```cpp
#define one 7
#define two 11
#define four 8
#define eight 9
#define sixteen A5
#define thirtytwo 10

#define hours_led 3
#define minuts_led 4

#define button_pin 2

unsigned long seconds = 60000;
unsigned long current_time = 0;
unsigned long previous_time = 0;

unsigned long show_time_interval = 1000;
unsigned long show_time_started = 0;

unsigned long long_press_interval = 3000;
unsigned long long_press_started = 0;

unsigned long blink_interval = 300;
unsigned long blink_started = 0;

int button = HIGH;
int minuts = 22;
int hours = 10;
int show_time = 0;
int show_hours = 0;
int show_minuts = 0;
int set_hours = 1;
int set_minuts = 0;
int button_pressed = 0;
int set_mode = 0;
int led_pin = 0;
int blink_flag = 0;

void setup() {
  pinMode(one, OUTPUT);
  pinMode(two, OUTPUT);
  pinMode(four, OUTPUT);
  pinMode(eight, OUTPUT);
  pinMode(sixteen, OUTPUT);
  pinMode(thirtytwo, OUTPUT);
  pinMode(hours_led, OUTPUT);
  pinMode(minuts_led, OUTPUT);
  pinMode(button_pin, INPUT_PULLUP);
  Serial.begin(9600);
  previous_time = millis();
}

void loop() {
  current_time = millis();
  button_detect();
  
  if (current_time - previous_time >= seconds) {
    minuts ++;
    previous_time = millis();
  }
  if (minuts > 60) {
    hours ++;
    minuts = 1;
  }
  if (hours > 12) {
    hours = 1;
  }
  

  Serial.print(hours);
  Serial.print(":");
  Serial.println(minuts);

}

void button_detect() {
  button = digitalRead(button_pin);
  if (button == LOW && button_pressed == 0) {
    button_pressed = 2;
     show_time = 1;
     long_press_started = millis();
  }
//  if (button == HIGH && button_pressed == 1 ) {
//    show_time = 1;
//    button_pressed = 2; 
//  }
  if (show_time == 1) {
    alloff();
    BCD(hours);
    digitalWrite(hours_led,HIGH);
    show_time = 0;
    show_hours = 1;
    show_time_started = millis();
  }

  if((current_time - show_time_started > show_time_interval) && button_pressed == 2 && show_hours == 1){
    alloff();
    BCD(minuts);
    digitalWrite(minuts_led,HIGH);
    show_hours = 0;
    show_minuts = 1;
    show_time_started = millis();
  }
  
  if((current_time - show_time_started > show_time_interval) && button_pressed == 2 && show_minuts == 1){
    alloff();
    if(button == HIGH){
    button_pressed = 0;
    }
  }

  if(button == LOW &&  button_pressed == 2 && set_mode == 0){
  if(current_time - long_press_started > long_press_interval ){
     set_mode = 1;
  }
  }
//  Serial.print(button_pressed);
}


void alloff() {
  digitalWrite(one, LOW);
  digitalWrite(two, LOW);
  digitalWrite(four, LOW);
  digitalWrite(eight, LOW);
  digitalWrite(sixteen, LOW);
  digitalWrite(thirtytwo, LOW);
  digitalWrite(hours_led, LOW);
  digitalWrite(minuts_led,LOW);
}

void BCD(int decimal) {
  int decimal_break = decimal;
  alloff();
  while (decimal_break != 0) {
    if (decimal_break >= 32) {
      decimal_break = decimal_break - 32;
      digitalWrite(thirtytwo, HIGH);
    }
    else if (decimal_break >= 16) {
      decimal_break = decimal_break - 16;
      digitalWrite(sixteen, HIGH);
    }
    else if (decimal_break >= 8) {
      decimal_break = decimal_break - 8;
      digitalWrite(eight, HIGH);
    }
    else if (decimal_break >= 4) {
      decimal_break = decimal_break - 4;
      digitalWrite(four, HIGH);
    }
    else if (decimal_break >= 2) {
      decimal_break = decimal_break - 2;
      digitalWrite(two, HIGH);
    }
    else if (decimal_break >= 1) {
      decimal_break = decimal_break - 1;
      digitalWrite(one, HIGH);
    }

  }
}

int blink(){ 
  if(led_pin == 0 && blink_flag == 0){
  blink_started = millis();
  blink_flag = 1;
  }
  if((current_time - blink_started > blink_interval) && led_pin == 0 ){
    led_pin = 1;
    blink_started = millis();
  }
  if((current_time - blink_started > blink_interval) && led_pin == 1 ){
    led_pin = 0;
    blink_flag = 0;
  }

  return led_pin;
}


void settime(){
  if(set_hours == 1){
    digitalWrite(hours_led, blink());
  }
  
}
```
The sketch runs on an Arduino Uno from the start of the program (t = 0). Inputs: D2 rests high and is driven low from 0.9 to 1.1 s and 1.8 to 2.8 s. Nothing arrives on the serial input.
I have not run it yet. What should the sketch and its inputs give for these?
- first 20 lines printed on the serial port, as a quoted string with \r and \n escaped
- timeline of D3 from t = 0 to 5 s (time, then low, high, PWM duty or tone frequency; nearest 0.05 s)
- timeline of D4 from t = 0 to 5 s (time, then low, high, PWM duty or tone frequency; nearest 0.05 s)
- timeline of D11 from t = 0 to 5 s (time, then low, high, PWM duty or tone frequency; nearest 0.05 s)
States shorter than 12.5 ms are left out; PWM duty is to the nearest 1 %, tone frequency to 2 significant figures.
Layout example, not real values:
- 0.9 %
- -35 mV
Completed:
- "10:22\r\n10:22\r\n10:22\r\n10:22\r\n10:22\r\n10:22\r\n10:22\r\n10:22\r\n10:22\r\n10:22\r\n10:22\r\n10:22\r\n10:22\r\n10:22\r\n10:22\r\n10:22\r\n10:22\r\n10:22\r\n10:22\r\n10:22\r\n"
- 0 s low; 0.9 s high; 1.9 s low
- 0 s low; 1.9 s high; 2.9 s low
- 0 s low; 0.9 s high; 2.9 s low
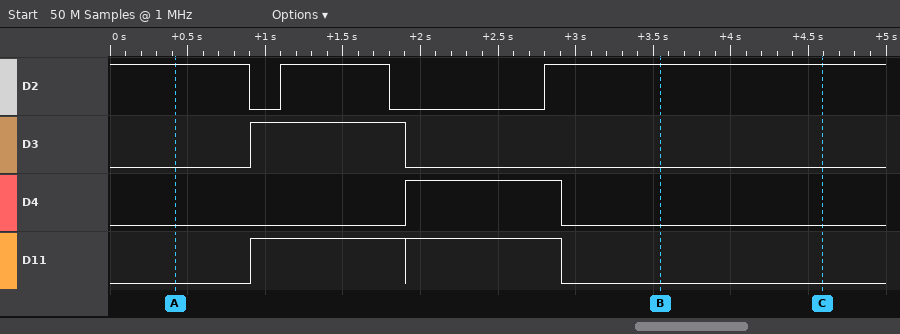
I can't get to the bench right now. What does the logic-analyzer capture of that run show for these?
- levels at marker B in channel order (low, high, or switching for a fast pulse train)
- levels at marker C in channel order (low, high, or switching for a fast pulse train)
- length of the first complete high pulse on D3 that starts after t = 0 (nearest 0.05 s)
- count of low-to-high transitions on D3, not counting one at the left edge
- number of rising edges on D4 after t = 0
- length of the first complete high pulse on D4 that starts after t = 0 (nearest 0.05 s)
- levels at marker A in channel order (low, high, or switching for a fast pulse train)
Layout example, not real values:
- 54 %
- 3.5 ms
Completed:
- D2 high, D3 low, D4 low, D11 low
- D2 high, D3 low, D4 low, D11 low
- 1.00 s
- 1
- 1
- 1.00 s
- D2 high, D3 low, D4 low, D11 low
